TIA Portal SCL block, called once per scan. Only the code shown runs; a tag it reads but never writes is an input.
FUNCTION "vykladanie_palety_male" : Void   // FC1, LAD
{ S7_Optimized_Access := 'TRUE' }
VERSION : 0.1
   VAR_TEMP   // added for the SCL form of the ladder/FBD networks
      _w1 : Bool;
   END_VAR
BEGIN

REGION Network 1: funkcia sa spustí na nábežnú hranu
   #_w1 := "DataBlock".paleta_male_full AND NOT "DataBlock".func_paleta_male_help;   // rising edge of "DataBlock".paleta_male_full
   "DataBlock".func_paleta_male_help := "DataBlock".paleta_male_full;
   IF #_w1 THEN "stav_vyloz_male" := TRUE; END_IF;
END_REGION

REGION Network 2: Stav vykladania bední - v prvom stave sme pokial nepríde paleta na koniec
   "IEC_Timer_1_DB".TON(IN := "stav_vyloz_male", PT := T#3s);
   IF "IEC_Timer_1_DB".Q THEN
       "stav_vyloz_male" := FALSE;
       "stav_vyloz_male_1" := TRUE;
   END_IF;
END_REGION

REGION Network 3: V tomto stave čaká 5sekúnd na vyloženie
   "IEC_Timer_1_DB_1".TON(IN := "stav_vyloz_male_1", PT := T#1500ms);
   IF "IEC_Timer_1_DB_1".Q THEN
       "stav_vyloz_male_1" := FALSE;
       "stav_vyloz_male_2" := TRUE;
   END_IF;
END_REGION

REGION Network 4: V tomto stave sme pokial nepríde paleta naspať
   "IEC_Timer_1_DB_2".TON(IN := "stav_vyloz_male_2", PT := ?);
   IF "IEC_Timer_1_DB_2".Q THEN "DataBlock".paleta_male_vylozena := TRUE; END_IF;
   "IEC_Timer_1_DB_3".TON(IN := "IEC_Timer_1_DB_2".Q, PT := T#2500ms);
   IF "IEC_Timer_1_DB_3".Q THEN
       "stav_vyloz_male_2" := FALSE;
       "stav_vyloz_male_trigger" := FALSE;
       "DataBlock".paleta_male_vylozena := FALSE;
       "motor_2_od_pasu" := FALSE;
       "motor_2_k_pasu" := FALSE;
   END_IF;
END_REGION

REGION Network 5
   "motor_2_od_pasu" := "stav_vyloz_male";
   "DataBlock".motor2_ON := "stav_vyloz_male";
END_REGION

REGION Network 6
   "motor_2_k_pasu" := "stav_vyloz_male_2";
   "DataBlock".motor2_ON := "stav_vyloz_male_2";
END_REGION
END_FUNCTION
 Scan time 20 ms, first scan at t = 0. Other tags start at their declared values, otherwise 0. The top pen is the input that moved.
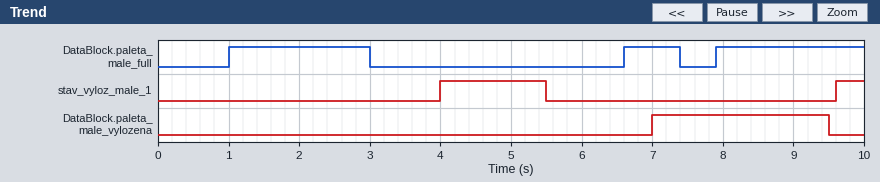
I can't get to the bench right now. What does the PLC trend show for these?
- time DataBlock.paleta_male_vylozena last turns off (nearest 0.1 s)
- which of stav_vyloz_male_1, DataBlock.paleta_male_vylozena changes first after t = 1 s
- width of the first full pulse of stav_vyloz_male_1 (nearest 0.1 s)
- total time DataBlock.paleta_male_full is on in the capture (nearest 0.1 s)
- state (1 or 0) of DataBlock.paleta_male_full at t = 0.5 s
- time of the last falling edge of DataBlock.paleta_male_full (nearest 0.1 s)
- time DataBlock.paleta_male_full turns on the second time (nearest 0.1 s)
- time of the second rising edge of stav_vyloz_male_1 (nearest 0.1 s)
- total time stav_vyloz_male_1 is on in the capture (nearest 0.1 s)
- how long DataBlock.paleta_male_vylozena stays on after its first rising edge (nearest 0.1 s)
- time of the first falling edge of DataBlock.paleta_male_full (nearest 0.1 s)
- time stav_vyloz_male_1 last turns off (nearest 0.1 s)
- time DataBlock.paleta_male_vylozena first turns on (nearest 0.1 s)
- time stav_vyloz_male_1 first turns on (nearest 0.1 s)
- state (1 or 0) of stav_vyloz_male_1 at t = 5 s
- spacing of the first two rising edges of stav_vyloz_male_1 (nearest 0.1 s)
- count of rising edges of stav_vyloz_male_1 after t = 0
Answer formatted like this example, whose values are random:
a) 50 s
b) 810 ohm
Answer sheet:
a) 9.5 s
b) stav_vyloz_male_1
c) 1.5 s
d) 4.9 s
e) 0
f) 7.4 s
g) 6.6 s
h) 9.6 s
i) 1.9 s
j) 2.5 s
k) 3.0 s
l) 5.5 s
m) 7.0 s
n) 4.0 s
o) 1
p) 5.6 s
q) 2
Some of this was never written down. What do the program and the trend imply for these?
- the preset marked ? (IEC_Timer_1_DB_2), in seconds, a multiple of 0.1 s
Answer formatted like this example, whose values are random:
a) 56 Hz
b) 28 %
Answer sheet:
a) 1.5 s
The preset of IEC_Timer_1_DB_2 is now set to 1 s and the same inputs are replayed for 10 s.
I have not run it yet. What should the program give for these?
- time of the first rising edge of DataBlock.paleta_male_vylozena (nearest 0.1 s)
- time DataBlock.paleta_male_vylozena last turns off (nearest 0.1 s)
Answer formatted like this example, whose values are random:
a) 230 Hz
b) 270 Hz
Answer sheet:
a) 6.5 s
b) 9.0 s
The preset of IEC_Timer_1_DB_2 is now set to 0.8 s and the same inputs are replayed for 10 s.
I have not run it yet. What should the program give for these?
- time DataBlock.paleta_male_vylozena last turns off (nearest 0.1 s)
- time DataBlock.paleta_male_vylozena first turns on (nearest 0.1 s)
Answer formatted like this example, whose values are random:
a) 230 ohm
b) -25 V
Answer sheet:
a) 8.8 s
b) 6.3 s
